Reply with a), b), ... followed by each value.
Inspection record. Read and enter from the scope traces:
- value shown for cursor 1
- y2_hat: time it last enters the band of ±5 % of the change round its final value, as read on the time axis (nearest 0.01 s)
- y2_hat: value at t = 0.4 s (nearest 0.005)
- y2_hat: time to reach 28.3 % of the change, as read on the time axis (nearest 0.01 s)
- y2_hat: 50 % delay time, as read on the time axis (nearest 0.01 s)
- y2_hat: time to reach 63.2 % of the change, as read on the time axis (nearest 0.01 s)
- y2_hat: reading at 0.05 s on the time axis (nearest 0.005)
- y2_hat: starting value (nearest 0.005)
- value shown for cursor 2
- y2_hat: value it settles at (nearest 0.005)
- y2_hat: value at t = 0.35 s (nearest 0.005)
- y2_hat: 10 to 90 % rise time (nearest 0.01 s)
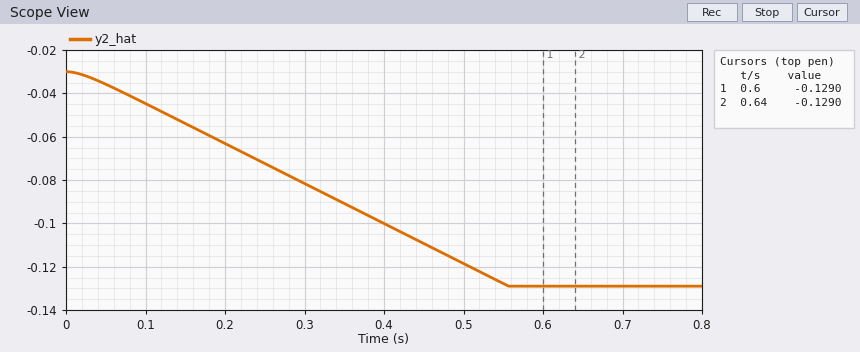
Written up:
a) -0.1290
b) 0.53 s
c) -0.100
d) 0.17 s
e) 0.29 s
f) 0.36 s
g) -0.035
h) -0.030
i) -0.1290
j) -0.130
k) -0.090
l) 0.43 s
